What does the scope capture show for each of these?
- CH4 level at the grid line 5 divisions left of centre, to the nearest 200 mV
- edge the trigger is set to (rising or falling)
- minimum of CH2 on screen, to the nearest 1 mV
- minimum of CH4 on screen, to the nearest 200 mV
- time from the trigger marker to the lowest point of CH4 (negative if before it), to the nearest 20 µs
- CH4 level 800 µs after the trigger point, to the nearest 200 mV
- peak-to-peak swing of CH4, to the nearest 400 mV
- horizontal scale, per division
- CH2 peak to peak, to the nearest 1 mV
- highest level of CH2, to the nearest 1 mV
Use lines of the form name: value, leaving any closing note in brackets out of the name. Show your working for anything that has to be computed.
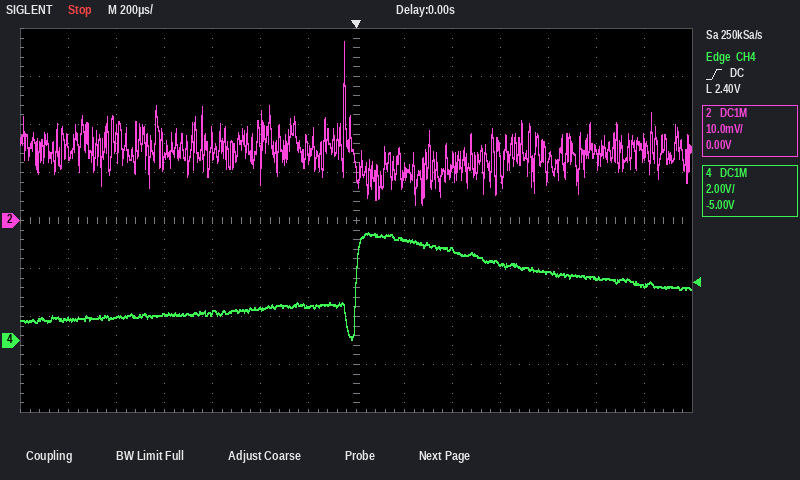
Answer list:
CH4 level at the grid line 5 divisions left of centre, to the nearest 200 mV: 1.0 V
edge the trigger is set to: rising
minimum of CH2 on screen, to the nearest 1 mV: 3 mV
minimum of CH4 on screen, to the nearest 200 mV: 0.0 V
time from the trigger marker to the lowest point of CH4 (negative if before it), to the nearest 20 µs: -20 µs
CH4 level 800 µs after the trigger point, to the nearest 200 mV: 2.8 V
peak-to-peak swing of CH4, to the nearest 400 mV: 4.4 V
horizontal scale, per division: 200 µs
CH2 peak to peak, to the nearest 1 mV: 37 mV − (3 mV) = 34 mV
highest level of CH2, to the nearest 1 mV: 37 mV
